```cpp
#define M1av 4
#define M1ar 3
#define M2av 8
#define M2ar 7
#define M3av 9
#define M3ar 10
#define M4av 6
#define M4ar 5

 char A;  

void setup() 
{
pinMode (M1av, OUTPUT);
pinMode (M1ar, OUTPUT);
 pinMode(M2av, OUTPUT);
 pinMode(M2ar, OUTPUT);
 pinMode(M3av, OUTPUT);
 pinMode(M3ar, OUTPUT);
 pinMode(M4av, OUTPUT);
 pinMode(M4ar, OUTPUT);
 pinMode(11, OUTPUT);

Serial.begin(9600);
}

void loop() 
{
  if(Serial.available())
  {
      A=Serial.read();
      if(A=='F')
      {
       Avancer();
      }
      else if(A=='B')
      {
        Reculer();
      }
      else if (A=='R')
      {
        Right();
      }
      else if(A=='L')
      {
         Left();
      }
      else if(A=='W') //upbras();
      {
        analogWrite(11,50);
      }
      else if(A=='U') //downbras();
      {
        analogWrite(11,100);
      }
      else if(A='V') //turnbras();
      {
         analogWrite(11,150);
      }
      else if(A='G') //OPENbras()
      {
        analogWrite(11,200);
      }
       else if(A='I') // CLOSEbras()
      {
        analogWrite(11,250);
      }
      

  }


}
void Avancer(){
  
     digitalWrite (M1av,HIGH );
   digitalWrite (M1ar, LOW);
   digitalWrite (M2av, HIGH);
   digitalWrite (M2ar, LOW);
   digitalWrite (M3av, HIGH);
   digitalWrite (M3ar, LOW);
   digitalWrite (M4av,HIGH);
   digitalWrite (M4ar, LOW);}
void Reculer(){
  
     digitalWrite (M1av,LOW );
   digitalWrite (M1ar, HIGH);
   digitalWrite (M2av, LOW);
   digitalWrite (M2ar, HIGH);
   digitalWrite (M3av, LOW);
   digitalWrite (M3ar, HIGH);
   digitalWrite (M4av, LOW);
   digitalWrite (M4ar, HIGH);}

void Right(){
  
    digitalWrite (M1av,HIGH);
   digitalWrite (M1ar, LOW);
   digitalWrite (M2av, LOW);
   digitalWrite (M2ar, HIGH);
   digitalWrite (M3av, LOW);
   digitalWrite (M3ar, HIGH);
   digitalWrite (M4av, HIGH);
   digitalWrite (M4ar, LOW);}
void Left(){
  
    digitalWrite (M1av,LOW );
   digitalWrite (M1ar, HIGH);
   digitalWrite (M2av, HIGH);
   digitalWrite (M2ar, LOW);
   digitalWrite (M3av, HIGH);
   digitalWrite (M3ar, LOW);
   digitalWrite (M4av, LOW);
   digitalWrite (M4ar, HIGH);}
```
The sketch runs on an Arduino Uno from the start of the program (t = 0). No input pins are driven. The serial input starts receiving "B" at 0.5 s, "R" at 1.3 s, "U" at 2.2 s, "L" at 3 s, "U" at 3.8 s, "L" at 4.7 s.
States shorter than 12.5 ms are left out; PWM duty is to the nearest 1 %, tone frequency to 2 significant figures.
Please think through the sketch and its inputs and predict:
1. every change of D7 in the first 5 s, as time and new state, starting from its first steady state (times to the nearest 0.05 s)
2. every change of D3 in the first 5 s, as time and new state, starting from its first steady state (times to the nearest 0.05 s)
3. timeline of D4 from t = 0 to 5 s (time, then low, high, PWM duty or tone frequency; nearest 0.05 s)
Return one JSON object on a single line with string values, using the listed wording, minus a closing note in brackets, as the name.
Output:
{"every change of D7 in the first 5 s, as time and new state, starting from its first steady state": "0 s low; 0.5 s high; 3 s low", "every change of D3 in the first 5 s, as time and new state, starting from its first steady state": "0 s low; 0.5 s high; 1.3 s low; 3 s high", "timeline of D4 from t = 0 to 5 s": "0 s low; 1.3 s high; 3 s low"}
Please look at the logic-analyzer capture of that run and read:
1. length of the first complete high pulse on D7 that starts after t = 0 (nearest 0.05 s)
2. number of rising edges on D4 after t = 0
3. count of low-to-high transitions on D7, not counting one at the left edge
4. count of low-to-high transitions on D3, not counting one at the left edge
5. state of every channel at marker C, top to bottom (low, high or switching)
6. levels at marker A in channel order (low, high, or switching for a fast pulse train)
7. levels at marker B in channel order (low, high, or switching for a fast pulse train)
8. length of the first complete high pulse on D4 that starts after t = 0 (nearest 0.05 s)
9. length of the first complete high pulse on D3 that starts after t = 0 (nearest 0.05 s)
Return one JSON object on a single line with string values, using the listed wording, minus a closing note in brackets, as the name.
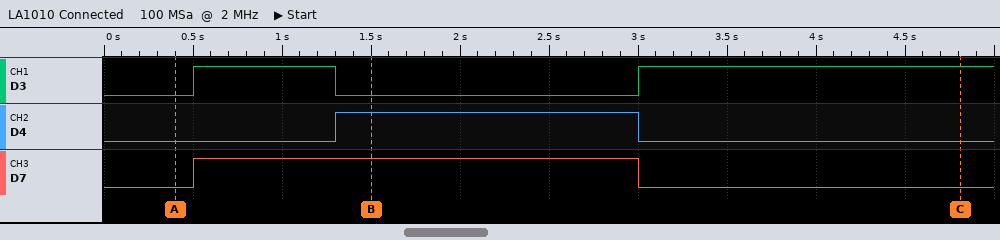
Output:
{"length of the first complete high pulse on D7 that starts after t = 0": "2.50 s", "number of rising edges on D4 after t = 0": "1", "count of low-to-high transitions on D7, not counting one at the left edge": "1", "count of low-to-high transitions on D3, not counting one at the left edge": "2", "state of every channel at marker C, top to bottom": "D3 high, D4 low, D7 low", "levels at marker A in channel order": "D3 low, D4 low, D7 low", "levels at marker B in channel order": "D3 low, D4 high, D7 high", "length of the first complete high pulse on D4 that starts after t = 0": "1.70 s", "length of the first complete high pulse on D3 that starts after t = 0": "0.80 s"}
